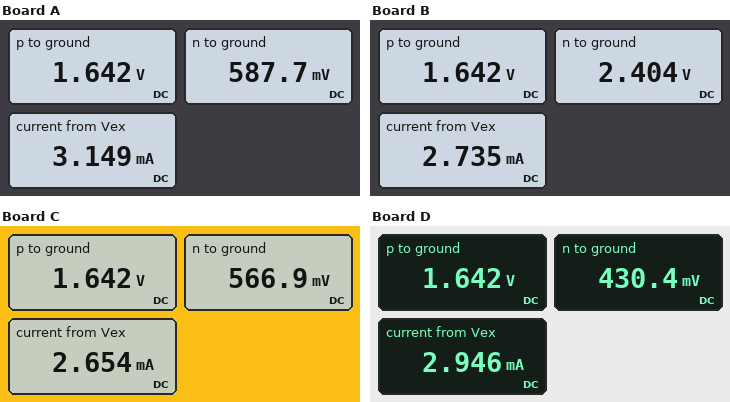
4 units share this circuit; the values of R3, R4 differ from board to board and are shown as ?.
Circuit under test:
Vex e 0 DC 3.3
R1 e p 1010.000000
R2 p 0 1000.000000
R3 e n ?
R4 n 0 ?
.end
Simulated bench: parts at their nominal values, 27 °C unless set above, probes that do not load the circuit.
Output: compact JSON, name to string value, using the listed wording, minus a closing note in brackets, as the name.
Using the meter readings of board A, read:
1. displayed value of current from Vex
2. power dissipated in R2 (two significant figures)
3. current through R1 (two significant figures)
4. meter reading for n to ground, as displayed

{"displayed value of current from Vex": "3.149 mA", "power dissipated in R2": "2.7 mW", "current through R1": "1.6 mA", "meter reading for n to ground, as displayed": "587.7 mV"}
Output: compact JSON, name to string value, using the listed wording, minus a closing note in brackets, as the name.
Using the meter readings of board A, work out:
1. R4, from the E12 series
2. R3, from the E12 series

{"R4, from the E12 series": "390 Ω", "R3, from the E12 series": "1.8 kΩ"}
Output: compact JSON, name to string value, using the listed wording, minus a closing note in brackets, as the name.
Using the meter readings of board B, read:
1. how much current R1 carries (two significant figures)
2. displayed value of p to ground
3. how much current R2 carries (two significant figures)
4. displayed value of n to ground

{"how much current R1 carries": "1.6 mA", "displayed value of p to ground": "1.642 V", "how much current R2 carries": "1.6 mA", "displayed value of n to ground": "2.404 V"}
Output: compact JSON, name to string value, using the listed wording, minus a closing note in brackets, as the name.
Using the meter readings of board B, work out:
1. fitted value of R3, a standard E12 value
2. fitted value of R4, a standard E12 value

{"fitted value of R3, a standard E12 value": "820 Ω", "fitted value of R4, a standard E12 value": "2.2 kΩ"}
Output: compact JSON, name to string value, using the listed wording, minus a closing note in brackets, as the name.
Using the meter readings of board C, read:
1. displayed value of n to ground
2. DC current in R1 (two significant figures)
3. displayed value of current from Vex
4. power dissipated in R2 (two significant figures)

{"displayed value of n to ground": "566.9 mV", "DC current in R1": "1.6 mA", "displayed value of current from Vex": "2.654 mA", "power dissipated in R2": "2.7 mW"}
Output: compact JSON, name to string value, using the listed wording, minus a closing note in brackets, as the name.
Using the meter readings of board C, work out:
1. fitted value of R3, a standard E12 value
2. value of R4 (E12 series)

{"fitted value of R3, a standard E12 value": "2.7 kΩ", "value of R4": "560 Ω"}
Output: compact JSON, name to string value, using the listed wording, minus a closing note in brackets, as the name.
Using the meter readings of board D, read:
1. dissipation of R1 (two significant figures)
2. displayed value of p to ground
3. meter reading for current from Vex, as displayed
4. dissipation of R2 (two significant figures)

{"dissipation of R1": "2.7 mW", "displayed value of p to ground": "1.642 V", "meter reading for current from Vex, as displayed": "2.946 mA", "dissipation of R2": "2.7 mW"}
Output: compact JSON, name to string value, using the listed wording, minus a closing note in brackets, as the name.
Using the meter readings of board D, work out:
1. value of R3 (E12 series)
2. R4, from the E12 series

{"value of R3": "2.2 kΩ", "R4, from the E12 series": "330 Ω"}
